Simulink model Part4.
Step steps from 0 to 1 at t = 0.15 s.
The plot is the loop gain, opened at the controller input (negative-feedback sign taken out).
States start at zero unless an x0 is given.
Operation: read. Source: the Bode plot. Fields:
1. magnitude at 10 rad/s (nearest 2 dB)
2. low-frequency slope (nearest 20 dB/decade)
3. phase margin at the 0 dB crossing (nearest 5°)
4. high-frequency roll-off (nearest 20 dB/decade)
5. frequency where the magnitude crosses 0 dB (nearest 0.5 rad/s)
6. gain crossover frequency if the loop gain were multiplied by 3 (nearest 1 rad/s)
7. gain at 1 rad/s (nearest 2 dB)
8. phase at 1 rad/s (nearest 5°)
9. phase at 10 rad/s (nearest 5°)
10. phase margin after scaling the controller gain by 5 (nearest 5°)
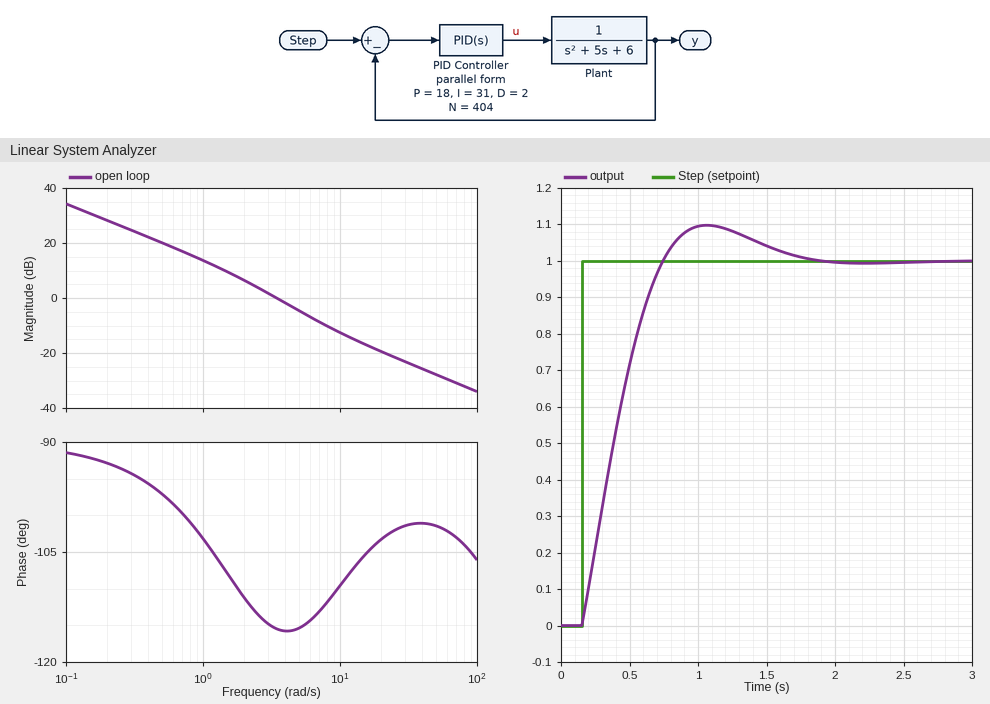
-12 dB
-20 dB/decade
65°
-20 dB/decade
3.5 rad/s
8 rad/s
14 dB
-105°
-110°
70°
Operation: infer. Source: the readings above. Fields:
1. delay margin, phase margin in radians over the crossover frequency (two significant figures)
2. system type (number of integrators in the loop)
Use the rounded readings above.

0.32 s
1
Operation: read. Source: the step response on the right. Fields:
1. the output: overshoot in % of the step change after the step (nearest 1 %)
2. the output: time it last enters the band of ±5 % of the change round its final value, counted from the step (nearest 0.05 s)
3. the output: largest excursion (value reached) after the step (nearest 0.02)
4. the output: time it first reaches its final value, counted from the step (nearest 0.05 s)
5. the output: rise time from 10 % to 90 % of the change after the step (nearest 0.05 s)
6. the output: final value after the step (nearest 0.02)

10 %
1.30 s
1.10
0.60 s
0.45 s
1.00
